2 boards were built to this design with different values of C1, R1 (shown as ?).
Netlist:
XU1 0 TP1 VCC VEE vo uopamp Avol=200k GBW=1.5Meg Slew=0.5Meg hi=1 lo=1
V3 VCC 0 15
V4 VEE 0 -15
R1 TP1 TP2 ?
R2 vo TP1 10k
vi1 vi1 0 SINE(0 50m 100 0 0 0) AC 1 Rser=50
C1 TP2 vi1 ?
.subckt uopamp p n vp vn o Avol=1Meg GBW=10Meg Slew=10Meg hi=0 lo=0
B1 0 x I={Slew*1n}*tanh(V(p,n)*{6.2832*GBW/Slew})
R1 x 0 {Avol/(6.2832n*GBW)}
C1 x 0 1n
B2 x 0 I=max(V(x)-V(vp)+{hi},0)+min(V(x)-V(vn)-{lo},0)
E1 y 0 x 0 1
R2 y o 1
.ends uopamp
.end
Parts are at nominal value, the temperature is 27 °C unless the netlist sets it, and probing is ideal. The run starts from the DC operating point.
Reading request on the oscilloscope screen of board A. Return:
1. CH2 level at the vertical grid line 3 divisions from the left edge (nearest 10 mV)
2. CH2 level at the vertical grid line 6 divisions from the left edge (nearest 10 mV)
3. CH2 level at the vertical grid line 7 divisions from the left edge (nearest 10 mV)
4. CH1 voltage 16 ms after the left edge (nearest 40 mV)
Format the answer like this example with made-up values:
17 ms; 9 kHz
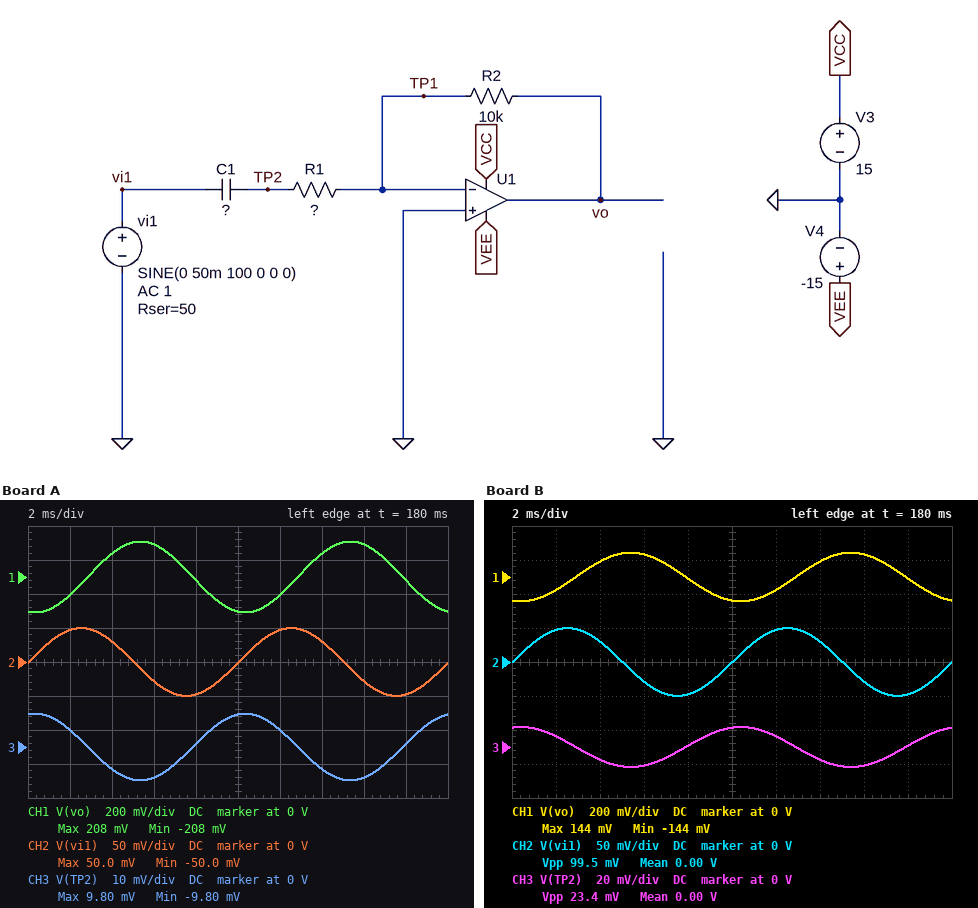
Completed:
-30 mV; 50 mV; 30 mV; 200 mV
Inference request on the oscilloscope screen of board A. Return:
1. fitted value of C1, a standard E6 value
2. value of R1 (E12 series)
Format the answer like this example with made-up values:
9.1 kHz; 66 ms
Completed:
680 nF; 470 Ω
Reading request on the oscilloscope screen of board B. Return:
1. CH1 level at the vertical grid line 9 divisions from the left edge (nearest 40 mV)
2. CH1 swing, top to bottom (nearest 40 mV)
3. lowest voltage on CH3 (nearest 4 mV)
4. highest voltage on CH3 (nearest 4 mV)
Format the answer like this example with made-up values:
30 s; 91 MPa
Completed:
0 V; 280 mV; -12 mV; 12 mV
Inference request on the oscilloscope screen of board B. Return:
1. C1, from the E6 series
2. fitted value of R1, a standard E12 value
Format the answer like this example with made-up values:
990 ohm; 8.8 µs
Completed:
470 nF; 820 Ω
